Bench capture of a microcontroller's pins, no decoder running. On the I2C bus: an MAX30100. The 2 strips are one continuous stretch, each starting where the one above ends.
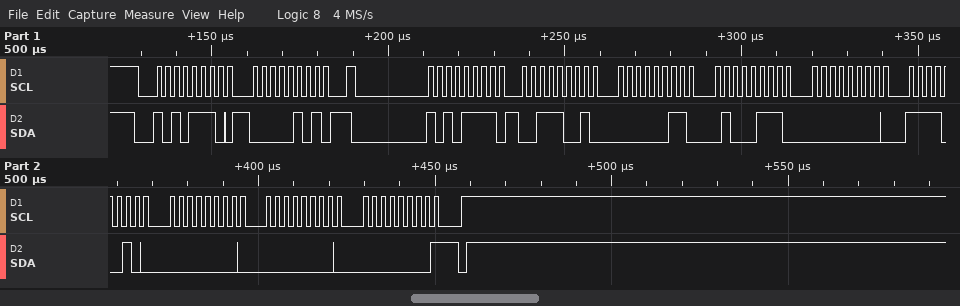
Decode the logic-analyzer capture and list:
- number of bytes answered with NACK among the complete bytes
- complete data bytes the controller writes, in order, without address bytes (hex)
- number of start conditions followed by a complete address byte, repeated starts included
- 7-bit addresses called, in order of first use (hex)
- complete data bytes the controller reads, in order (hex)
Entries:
1
05
2
0x57
39 03 47 00 F2 00 00 00
